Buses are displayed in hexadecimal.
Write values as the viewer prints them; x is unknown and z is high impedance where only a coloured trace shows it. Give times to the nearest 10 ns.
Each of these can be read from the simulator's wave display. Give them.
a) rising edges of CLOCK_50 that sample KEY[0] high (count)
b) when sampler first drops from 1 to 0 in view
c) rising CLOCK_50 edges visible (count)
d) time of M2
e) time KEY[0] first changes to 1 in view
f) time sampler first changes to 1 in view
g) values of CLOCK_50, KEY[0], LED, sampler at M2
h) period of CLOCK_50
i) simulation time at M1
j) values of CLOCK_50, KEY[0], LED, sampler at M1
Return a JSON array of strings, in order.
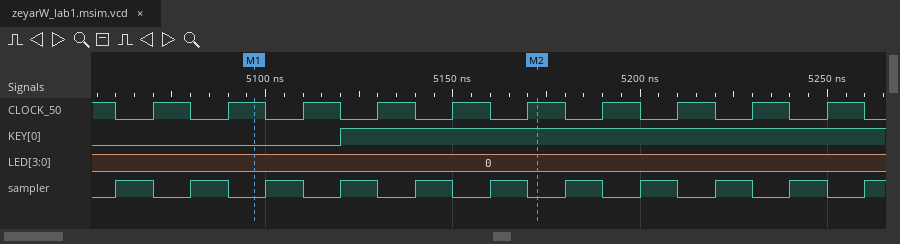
["7", "5070 ns", "10", "5170 ns", "5120 ns", "5060 ns", "CLOCK_50=1, KEY[0]=1, LED=0, sampler=0", "20 ns", "5100 ns", "CLOCK_50=1, KEY[0]=0, LED=0, sampler=0"]
